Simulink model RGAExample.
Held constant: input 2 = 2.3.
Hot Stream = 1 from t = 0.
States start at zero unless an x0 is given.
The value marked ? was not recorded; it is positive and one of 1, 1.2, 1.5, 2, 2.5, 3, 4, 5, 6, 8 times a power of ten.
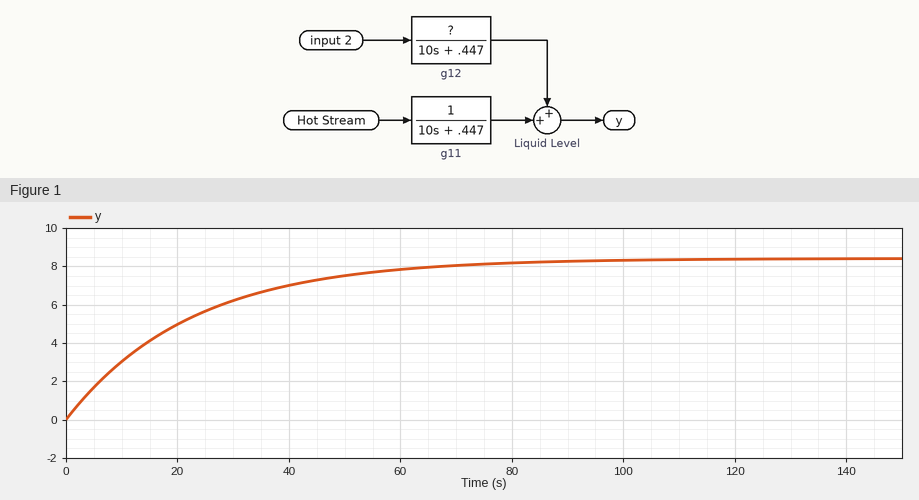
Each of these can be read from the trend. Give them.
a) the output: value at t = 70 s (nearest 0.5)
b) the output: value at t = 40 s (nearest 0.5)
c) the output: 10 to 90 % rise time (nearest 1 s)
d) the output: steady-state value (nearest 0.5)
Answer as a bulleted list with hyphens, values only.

- 8.0
- 7.0
- 49 s
- 8.5
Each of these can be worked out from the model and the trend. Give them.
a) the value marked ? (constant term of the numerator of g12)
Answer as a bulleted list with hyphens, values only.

- 1.2
